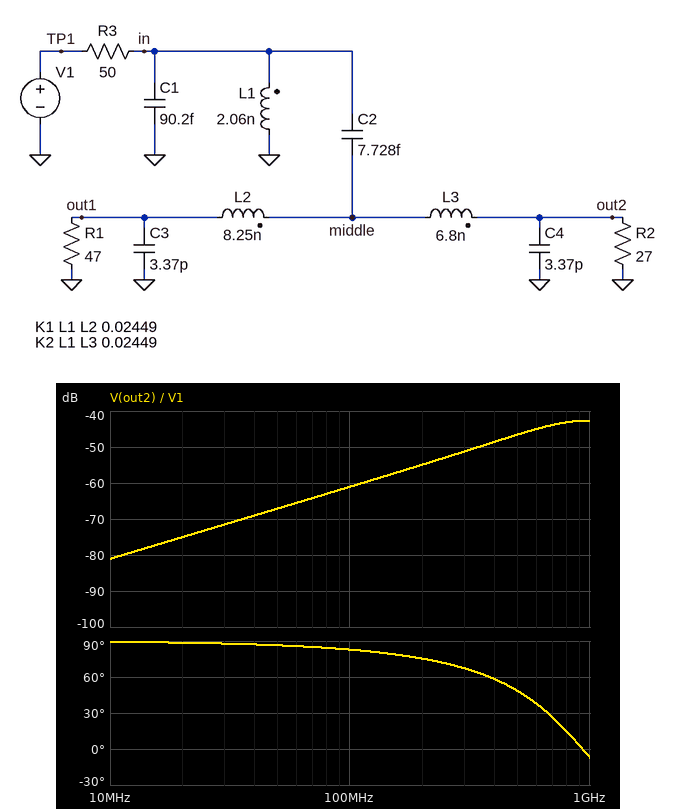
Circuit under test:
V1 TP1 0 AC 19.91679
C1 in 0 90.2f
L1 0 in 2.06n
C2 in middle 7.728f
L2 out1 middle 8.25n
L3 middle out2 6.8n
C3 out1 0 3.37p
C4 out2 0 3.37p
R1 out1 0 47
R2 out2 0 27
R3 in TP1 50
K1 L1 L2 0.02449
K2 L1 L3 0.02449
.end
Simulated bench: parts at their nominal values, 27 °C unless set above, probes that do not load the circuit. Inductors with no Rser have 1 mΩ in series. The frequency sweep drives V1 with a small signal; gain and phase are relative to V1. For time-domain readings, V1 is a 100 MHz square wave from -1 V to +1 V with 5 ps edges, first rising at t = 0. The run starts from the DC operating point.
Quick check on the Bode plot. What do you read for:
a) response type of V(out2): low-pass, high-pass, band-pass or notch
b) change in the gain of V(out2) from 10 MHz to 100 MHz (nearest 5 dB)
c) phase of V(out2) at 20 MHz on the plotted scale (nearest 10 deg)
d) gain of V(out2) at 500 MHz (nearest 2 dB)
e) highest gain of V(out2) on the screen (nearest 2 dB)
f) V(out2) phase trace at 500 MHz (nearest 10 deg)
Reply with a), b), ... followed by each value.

a) high-pass
b) 20 dB
c) 90 deg
d) -46 dB
e) -42 dB
f) 50 deg
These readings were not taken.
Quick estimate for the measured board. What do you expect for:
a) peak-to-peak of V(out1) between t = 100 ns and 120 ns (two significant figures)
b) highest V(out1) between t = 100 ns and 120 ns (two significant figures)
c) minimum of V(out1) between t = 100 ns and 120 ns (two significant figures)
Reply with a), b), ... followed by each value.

a) 28 mV
b) 14 mV
c) -14 mV
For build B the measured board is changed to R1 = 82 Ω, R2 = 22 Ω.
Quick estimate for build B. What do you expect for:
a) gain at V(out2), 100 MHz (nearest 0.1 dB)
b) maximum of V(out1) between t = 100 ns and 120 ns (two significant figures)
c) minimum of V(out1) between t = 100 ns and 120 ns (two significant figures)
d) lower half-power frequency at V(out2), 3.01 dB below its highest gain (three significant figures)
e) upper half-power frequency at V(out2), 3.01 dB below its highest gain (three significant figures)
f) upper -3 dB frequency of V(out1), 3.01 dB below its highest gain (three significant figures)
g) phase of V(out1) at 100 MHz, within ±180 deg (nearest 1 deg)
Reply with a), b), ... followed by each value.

a) -65.6 dB
b) 18 mV
c) -18 mV
d) 615 MHz
e) 1.60 GHz
f) 1.30 GHz
g) -98 deg
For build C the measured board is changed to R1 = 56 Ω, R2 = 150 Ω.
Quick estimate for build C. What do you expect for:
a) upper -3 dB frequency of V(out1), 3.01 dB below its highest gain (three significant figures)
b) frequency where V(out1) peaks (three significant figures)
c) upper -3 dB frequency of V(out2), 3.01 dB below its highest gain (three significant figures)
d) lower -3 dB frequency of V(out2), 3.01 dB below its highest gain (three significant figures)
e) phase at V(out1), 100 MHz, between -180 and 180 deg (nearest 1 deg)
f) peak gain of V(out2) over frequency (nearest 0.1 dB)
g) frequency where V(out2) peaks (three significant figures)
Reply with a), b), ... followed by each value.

a) 1.30 GHz
b) 979 MHz
c) 1.23 GHz
d) 709 MHz
e) -87 deg
f) -32.3 dB
g) 948 MHz
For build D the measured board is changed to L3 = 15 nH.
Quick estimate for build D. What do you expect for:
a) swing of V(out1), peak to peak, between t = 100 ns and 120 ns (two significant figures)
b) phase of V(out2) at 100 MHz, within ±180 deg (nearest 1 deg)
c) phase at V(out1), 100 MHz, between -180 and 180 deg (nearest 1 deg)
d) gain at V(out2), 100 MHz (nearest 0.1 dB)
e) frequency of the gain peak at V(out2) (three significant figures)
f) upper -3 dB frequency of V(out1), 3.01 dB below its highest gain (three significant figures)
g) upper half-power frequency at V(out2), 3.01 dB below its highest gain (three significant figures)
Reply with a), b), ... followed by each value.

a) 26 mV
b) 79 deg
c) -104 deg
d) -59.3 dB
e) 811 MHz
f) 1.51 GHz
g) 1.66 GHz
